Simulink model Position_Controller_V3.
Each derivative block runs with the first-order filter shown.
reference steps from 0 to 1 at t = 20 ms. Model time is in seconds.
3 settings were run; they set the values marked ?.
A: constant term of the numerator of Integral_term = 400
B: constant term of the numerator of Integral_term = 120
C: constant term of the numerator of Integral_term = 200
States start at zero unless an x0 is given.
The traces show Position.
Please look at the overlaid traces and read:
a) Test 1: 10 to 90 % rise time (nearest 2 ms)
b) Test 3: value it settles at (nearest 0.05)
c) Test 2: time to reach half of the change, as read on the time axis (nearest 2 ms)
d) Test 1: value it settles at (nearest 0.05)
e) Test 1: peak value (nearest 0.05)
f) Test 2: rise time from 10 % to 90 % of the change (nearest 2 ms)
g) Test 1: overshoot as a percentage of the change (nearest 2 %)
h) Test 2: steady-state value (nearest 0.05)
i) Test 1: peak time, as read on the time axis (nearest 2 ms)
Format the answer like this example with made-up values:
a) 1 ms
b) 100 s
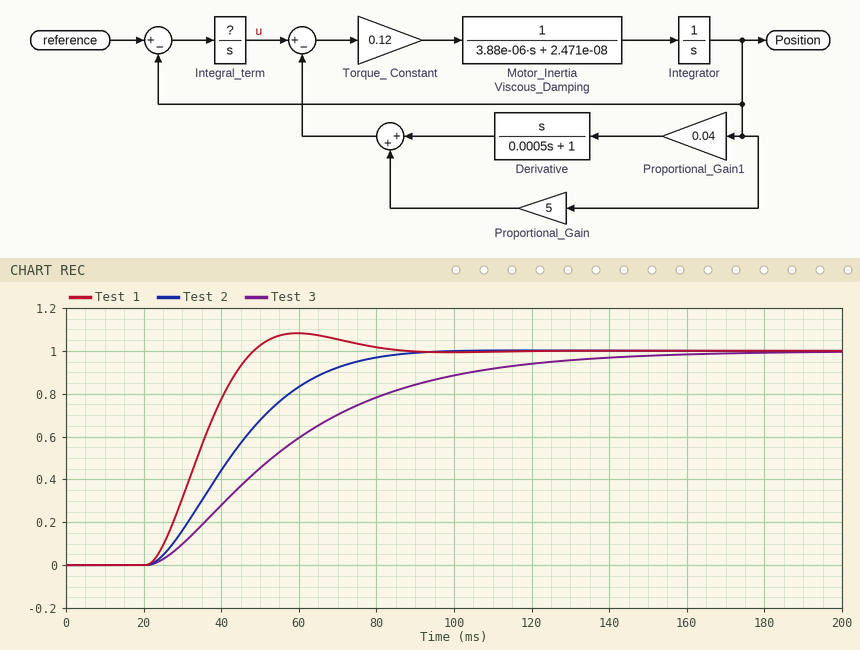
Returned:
a) 18 ms
b) 1.00
c) 42 ms
d) 1.00
e) 1.10
f) 40 ms
g) 8 %
h) 1.00
i) 60 ms
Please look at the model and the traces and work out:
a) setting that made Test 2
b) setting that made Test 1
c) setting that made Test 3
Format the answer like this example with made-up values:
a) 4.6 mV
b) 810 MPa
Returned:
a) C
b) A
c) B
